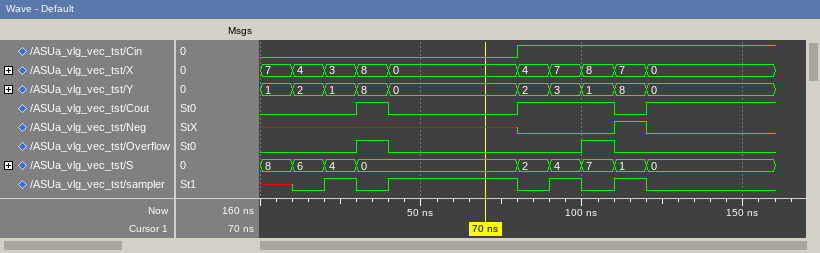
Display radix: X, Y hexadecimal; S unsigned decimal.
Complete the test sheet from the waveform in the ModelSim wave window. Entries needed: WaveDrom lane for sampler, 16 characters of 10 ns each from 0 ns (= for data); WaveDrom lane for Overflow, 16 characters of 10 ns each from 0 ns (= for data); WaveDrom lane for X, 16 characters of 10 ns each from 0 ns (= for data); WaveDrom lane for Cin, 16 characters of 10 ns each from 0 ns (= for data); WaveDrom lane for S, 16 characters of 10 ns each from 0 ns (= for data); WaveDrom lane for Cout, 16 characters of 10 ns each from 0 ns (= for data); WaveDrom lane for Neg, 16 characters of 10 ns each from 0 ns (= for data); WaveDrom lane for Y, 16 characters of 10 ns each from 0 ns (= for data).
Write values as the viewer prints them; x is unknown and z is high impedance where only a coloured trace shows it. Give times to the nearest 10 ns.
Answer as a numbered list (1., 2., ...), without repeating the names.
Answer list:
1. {name: 'sampler', wave: 'x0101...01010...'}
2. {name: 'Overflow', wave: '0..10.....10....'}
3. {name: 'X', wave: '=====...=====...', data: '7 4 3 8 0 4 7 8 7 0'}
4. {name: 'Cin', wave: '0.......1.......'}
5. {name: 'S', wave: '====....=====...', data: '8 6 4 0 2 4 7 1 0'}
6. {name: 'Cout', wave: '0..10...1..01...'}
7. {name: 'Neg', wave: 'x.......0..10...'}
8. {name: 'Y', wave: '=====...=====...', data: '1 2 1 8 0 2 3 1 8 0'}
